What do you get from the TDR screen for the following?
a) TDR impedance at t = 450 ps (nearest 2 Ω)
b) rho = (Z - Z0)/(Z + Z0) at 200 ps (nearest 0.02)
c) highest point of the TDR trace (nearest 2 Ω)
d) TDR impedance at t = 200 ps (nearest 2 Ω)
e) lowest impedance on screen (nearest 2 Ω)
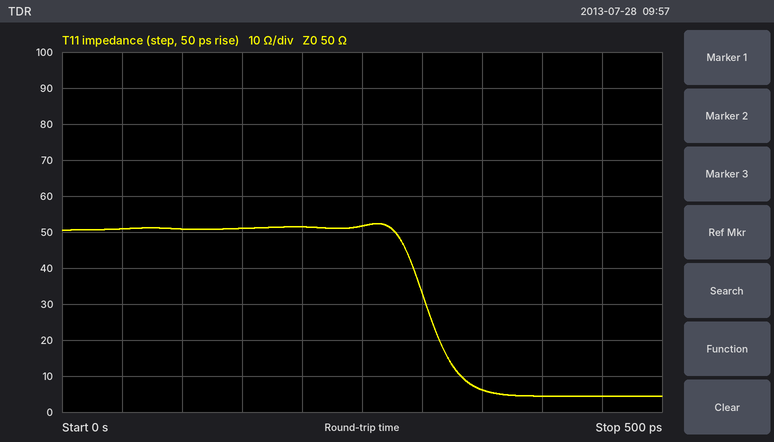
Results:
4 Ω
+0.02
52 Ω
52 Ω
4 Ω
